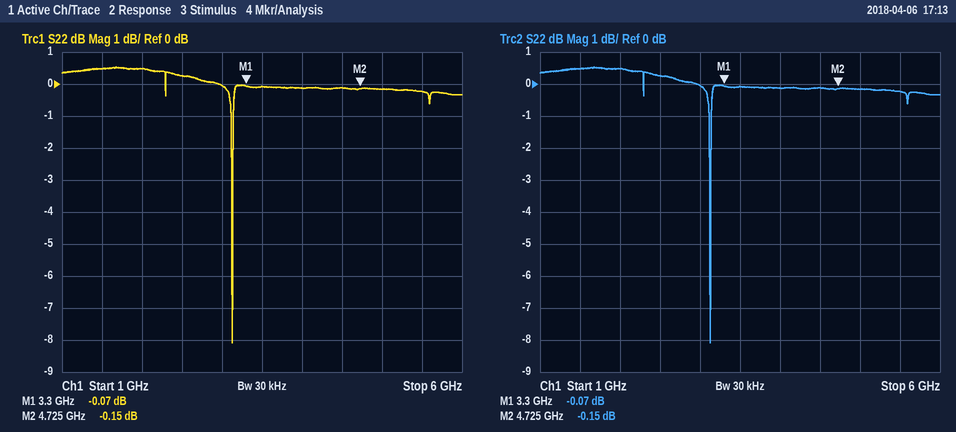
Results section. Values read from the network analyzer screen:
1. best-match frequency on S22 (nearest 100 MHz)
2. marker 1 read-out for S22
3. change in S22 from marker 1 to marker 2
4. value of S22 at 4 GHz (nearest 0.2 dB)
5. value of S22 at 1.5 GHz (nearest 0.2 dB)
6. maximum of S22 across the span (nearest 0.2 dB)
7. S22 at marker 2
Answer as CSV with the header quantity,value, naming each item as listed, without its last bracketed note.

quantity,value
best-match frequency on S22,3.1 GHz
marker 1 read-out for S22,-0.07 dB
change in S22 from marker 1 to marker 2,-0.08 dB
value of S22 at 4 GHz,-0.2 dB
value of S22 at 1.5 GHz,0.4 dB
maximum of S22 across the span,0.6 dB
S22 at marker 2,-0.15 dB
